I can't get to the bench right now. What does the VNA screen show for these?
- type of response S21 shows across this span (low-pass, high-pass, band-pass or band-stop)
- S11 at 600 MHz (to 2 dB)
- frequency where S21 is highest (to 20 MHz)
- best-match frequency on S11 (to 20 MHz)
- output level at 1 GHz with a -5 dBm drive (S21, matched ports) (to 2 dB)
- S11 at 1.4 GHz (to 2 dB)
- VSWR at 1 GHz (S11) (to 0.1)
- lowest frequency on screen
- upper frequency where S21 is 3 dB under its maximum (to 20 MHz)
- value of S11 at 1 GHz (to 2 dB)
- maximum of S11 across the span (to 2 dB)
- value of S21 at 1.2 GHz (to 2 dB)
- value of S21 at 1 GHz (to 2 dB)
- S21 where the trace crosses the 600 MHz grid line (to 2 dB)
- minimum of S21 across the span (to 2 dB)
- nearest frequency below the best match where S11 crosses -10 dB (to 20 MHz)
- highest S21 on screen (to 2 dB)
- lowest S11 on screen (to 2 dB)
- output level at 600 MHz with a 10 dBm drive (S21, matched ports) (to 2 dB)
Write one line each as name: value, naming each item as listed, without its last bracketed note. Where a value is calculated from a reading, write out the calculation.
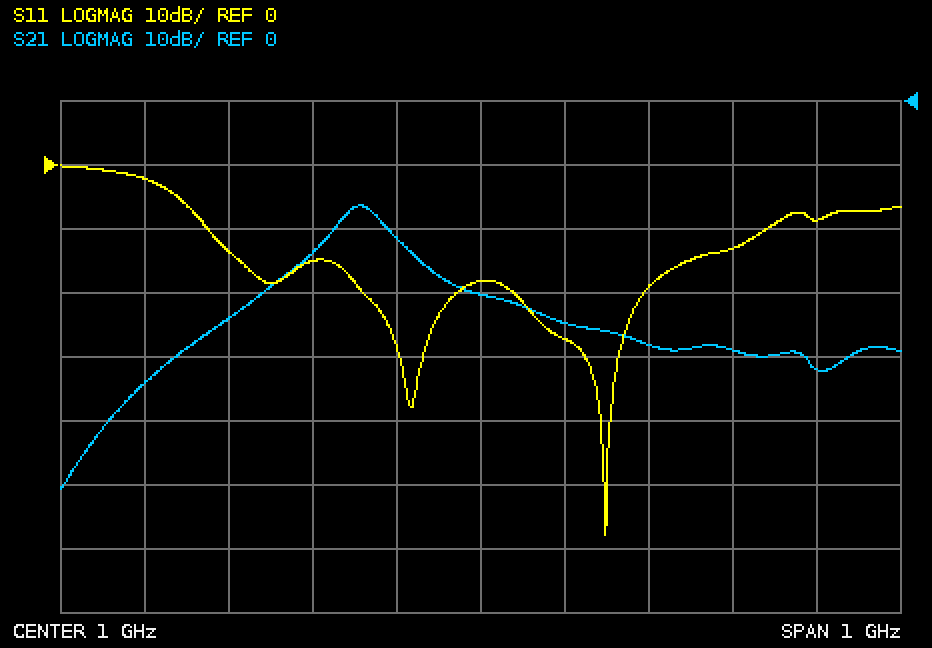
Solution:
type of response S21 shows across this span: band-pass
S11 at 600 MHz: -2 dB
frequency where S21 is highest: 860 MHz
best-match frequency on S11: 1.14 GHz
output level at 1 GHz with a -5 dBm drive (S21, matched ports): -5 dBm + (-30 dB) = -36 dBm
S11 at 1.4 GHz: -8 dB
VSWR at 1 GHz (S11): |Γ| = 10^(-18/20) = 0.1259; VSWR = (1 + 0.1259)/(1 − 0.1259) ≈ 1.3
lowest frequency on screen: 500 MHz
upper frequency where S21 is 3 dB under its maximum: 880 MHz
value of S11 at 1 GHz: -18 dB
maximum of S11 across the span: 0 dB
value of S21 at 1.2 GHz: -38 dB
value of S21 at 1 GHz: -30 dB
S21 where the trace crosses the 600 MHz grid line: -44 dB
minimum of S21 across the span: -60 dB
nearest frequency below the best match where S11 crosses -10 dB: 680 MHz
highest S21 on screen: -16 dB
lowest S11 on screen: -58 dB
output level at 600 MHz with a 10 dBm drive (S21, matched ports): 10 dBm + (-44 dB) = -34 dBm
